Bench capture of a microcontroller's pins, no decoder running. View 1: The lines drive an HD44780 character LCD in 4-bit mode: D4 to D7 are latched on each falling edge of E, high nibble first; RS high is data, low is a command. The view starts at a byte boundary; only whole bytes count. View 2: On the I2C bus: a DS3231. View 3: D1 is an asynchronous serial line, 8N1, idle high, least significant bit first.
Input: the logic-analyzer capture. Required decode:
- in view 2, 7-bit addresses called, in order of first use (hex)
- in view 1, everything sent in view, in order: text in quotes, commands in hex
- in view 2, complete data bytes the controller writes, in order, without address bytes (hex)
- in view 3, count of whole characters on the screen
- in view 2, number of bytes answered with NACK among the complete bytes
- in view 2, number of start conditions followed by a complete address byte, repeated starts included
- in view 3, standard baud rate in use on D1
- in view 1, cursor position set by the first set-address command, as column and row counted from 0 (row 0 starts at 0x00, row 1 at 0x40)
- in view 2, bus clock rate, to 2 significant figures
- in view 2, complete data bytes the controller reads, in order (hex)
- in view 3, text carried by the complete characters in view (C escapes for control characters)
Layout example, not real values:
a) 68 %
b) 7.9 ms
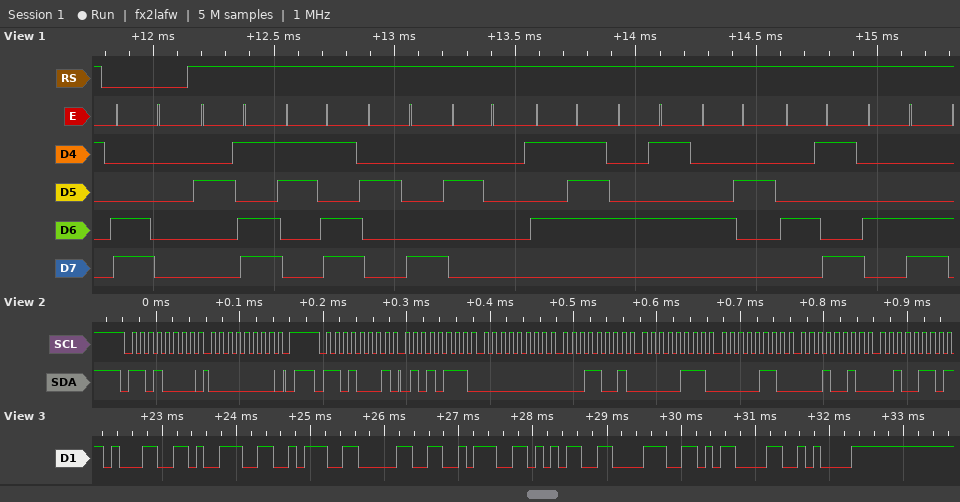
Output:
a) 0x68
b) 0xC0 "-=( WEBIL"
c) 00
d) 9
e) 1
f) 2
g) 9600 baud
h) column 0, row 1
i) 100 kHz
j) 57 00 19 07 06 12 26
k) "19:0:58\r\n"
